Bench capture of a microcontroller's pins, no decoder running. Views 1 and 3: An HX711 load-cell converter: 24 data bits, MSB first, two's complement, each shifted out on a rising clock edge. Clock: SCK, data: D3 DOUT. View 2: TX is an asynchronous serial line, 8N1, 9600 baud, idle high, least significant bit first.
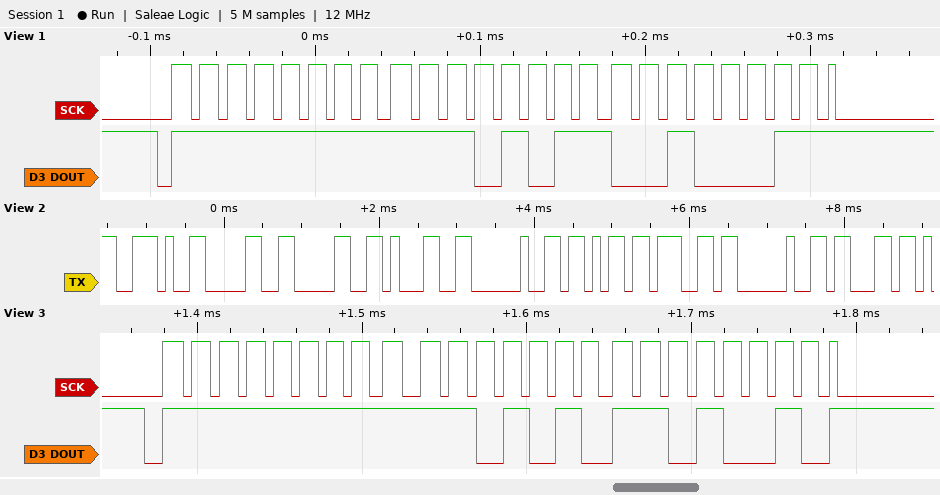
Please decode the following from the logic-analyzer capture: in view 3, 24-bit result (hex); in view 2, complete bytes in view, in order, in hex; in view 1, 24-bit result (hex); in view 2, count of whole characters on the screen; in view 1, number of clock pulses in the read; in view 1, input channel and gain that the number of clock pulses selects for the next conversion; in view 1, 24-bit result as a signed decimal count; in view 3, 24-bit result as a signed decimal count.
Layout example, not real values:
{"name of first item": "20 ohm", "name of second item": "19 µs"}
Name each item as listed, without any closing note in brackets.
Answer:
{"in view 3, 24-bit result": "0xFFEAD2", "in view 2, complete bytes in view, in order, in hex": "2E 30 30 31 20 6B 67 20 63", "in view 1, 24-bit result": "0xFFEB23", "in view 2, count of whole characters on the screen": "9", "in view 1, number of clock pulses in the read": "25", "in view 1, input channel and gain that the number of clock pulses selects for the next conversion": "channel A, gain 128", "in view 1, 24-bit result as a signed decimal count": "-5341", "in view 3, 24-bit result as a signed decimal count": "-5422"}
